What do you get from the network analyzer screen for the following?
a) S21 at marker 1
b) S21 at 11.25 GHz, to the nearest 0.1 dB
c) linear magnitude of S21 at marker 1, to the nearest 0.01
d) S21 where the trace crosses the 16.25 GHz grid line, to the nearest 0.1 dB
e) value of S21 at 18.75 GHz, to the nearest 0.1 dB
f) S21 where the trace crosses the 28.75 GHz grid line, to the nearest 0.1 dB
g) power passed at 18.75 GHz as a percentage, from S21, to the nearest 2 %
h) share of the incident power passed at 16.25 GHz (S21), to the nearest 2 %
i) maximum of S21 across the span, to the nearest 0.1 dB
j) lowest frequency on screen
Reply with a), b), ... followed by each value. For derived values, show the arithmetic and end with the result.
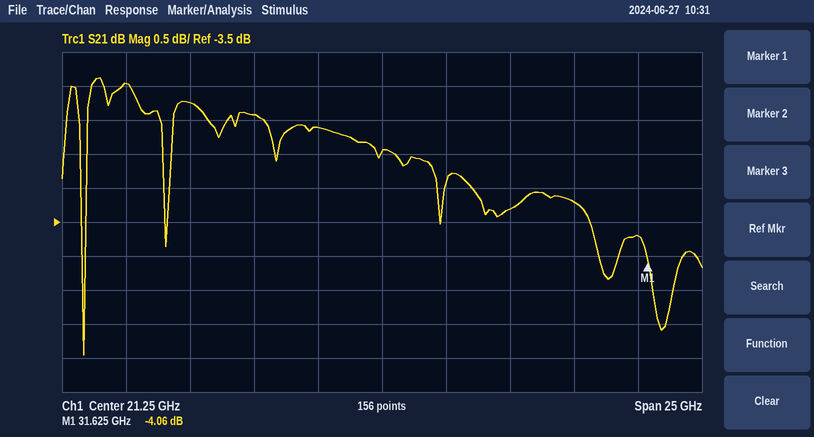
a) -4.06 dB
b) -1.5 dB
c) 10^(-4.06/20) ≈ 0.63
d) -1.9 dB
e) -2.1 dB
f) -3.2 dB
g) 10^(-2.1/10) ≈ 62 %
h) 10^(-1.9/10) ≈ 64.6 %, so 64 % to the nearest 2 %
i) -1.4 dB
j) 8.75 GHz
